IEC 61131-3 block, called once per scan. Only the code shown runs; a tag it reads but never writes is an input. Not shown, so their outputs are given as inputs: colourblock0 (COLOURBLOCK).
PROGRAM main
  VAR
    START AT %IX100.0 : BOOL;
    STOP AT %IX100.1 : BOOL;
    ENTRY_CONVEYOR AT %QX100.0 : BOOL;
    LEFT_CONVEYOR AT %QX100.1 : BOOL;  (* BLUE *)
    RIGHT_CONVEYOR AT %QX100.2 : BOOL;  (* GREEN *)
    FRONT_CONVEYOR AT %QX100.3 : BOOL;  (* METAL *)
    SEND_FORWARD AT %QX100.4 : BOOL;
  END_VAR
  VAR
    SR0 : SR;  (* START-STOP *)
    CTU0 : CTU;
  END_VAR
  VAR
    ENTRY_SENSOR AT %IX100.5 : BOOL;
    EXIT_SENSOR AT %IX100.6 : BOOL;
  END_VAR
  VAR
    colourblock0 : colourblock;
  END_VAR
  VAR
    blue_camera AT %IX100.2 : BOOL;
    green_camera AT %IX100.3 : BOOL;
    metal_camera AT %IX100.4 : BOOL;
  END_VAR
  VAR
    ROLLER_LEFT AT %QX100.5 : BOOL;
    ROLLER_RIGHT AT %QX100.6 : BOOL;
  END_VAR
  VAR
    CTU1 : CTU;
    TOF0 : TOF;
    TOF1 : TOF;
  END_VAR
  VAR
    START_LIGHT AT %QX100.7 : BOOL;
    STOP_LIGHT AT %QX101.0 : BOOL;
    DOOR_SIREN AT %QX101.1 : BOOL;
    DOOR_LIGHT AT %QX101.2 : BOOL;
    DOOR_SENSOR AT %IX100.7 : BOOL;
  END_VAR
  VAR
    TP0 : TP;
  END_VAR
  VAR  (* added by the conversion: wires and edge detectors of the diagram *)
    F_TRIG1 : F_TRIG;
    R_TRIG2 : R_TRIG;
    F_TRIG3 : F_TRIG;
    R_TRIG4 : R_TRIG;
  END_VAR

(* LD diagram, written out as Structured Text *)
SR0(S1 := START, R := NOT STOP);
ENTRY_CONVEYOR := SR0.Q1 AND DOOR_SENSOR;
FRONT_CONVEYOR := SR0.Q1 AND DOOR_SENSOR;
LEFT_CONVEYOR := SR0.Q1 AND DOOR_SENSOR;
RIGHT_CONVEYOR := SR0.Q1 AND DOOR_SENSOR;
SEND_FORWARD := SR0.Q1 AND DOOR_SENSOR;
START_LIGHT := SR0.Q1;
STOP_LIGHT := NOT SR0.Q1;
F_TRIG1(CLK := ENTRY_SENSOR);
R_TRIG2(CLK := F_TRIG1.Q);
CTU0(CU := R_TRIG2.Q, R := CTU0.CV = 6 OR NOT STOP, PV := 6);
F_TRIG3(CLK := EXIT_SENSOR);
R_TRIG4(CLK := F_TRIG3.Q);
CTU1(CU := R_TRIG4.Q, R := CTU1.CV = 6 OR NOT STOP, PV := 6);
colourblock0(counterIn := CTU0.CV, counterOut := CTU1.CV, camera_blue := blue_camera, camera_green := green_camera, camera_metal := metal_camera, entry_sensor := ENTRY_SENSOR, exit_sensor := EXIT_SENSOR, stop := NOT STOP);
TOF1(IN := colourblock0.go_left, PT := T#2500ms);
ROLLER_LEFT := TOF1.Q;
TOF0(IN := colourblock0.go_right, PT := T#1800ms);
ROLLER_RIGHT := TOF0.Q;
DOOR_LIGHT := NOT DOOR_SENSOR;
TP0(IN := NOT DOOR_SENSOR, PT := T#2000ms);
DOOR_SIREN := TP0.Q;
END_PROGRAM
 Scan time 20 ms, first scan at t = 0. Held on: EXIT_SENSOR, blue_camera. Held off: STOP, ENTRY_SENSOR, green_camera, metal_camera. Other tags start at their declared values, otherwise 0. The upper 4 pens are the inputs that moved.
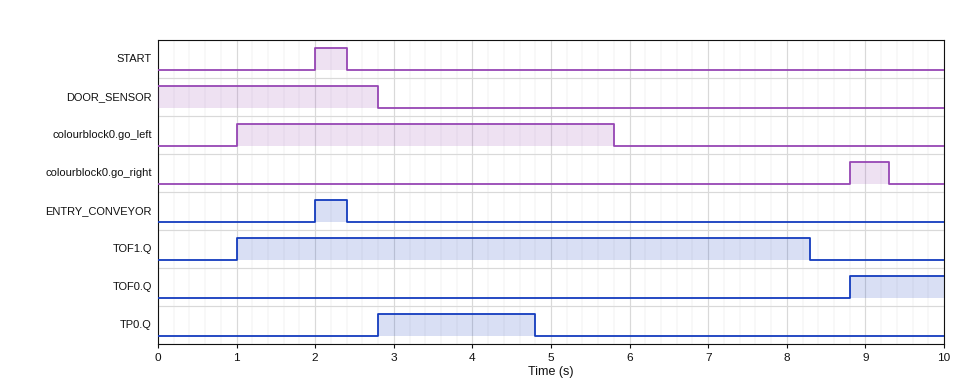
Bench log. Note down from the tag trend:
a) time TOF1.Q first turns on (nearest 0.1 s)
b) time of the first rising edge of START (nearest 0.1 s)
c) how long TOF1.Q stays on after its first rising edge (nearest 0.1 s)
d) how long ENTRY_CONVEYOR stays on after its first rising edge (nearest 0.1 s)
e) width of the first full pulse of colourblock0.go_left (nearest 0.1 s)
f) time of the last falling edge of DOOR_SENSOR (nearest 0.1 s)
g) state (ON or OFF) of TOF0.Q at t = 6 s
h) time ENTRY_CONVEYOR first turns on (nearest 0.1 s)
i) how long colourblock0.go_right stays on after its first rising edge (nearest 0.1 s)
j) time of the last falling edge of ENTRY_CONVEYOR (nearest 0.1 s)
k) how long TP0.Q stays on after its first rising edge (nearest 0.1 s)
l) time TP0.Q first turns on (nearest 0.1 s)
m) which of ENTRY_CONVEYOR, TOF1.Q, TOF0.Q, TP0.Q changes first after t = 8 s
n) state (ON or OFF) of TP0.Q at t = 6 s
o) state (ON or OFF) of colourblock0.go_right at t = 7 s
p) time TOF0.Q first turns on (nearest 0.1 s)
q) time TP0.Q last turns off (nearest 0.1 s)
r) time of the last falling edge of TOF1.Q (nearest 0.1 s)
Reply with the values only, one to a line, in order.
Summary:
1.0 s
2.0 s
7.3 s
0.4 s
4.8 s
2.8 s
OFF
2.0 s
0.5 s
2.4 s
2.0 s
2.8 s
TOF1.Q
OFF
OFF
8.8 s
4.8 s
8.3 s
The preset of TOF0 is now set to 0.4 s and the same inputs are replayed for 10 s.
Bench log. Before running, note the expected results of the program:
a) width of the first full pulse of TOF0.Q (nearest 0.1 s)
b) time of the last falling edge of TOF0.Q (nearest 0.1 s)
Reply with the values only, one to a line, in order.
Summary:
0.9 s
9.7 s
